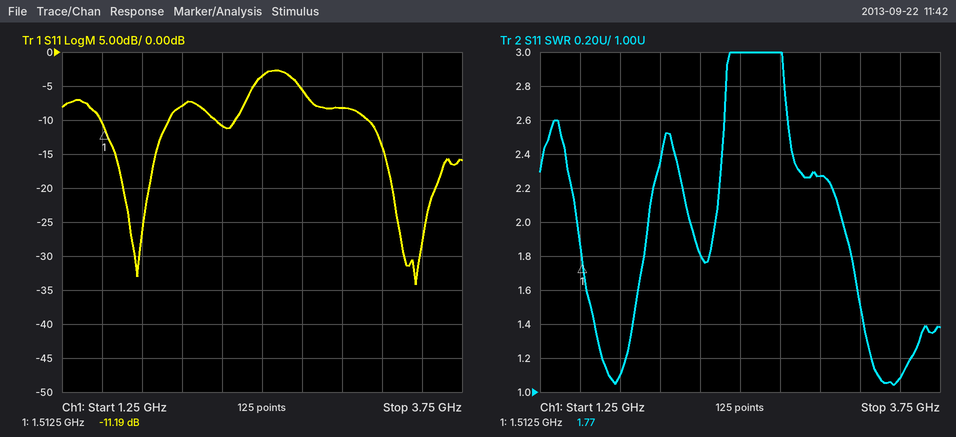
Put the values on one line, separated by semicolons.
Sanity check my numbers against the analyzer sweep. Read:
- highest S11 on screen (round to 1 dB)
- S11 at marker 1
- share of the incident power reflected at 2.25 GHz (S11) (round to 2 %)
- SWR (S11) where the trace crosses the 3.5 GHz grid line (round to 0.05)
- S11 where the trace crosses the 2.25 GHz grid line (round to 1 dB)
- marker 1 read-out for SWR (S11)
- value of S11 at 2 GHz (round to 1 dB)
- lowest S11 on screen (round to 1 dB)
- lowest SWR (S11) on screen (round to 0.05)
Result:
-3 dB; -11.19 dB; 8 %; 1.10; -11 dB; 1.77; -8 dB; -34 dB; 1.05
